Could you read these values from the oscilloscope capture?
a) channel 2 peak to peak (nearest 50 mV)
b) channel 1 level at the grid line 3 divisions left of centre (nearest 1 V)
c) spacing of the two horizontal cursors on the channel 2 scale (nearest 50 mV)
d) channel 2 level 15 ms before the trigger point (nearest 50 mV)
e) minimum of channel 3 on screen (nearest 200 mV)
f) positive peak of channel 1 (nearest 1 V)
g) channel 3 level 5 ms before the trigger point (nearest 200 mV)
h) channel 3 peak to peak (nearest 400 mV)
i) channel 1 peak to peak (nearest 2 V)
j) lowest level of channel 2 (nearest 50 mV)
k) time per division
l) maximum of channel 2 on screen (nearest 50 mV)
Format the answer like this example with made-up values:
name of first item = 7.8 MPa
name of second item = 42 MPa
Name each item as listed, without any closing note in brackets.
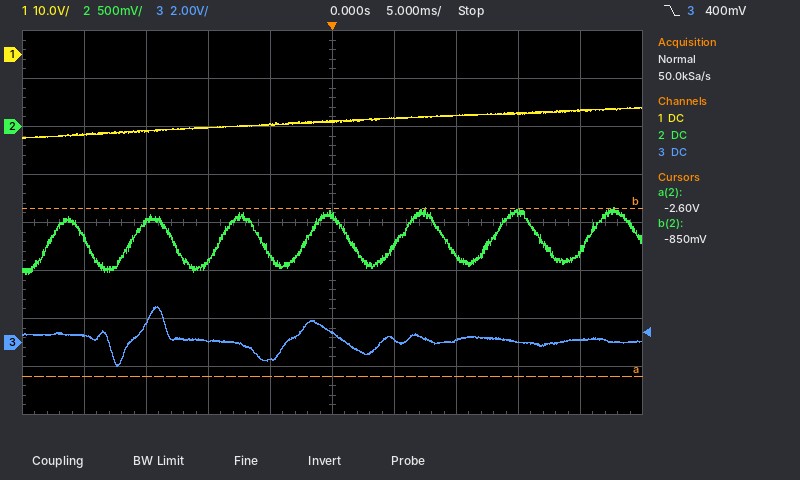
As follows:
channel 2 peak to peak = 700 mV
channel 1 level at the grid line 3 divisions left of centre = -16 V
spacing of the two horizontal cursors on the channel 2 scale = 1.75 V
channel 2 level 15 ms before the trigger point = -1.00 V
minimum of channel 3 on screen = -1.0 V
positive peak of channel 1 = -11 V
channel 3 level 5 ms before the trigger point = -800 mV
channel 3 peak to peak = 2.4 V
channel 1 peak to peak = 6 V
lowest level of channel 2 = -1.55 V
time per division = 5 ms
maximum of channel 2 on screen = -850 mV
